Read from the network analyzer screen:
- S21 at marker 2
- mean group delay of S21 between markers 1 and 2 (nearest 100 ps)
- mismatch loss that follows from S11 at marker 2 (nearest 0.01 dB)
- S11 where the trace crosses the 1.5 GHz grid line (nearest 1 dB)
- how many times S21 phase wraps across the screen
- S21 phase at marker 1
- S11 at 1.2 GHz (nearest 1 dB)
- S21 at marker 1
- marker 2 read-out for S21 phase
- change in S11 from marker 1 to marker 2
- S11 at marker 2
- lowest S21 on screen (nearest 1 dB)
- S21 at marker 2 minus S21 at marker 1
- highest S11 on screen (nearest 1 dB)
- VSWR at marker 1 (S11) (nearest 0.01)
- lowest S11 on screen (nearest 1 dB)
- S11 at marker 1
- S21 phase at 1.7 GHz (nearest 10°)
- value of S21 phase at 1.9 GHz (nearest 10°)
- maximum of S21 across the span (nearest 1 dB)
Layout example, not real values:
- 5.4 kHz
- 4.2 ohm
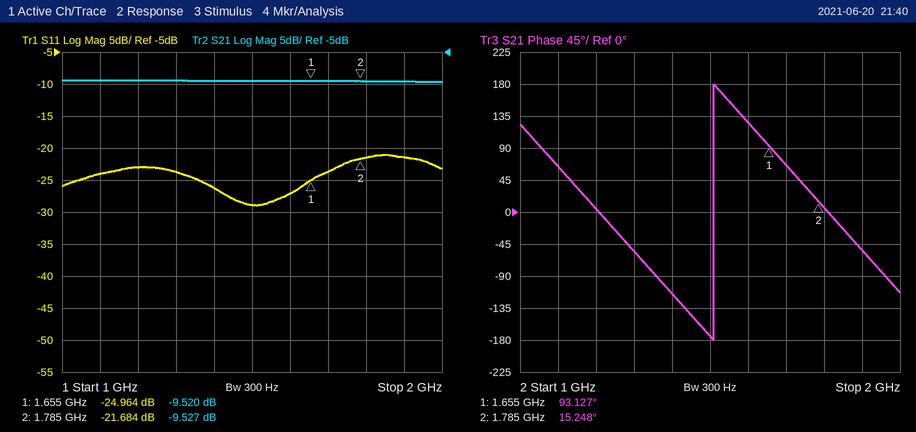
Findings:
- -9.527 dB
- 1.7 ns
- 0.03 dB
- -29 dB
- 1
- 93.127°
- -23 dB
- -9.520 dB
- 15.248°
- 3.280 dB
- -21.684 dB
- -10 dB
- -0.007 dB
- -21 dB
- 1.12
- -29 dB
- -24.964 dB
- 70°
- -50°
- -9 dB
